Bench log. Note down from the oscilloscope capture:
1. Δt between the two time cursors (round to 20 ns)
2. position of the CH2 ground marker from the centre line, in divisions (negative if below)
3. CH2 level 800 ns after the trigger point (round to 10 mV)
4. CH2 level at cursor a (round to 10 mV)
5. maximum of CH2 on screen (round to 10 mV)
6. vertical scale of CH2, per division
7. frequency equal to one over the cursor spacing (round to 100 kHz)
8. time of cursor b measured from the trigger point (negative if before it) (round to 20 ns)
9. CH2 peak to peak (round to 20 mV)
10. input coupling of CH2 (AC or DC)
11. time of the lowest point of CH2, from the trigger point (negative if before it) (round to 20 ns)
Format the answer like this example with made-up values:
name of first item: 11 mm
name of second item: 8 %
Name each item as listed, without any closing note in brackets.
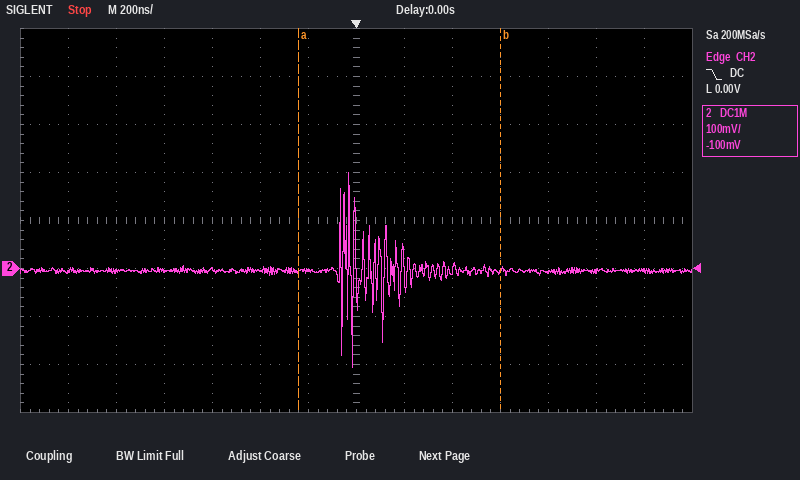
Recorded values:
Δt between the two time cursors: 840 ns
position of the CH2 ground marker from the centre line, in divisions: -1.0 div
CH2 level 800 ns after the trigger point: -10 mV
CH2 level at cursor a: -10 mV
maximum of CH2 on screen: 200 mV
vertical scale of CH2, per division: 100 mV
frequency equal to one over the cursor spacing: 1.2 MHz
time of cursor b measured from the trigger point (negative if before it): +600 ns
CH2 peak to peak: 400 mV
input coupling of CH2: DC
time of the lowest point of CH2, from the trigger point (negative if before it): -20 ns
